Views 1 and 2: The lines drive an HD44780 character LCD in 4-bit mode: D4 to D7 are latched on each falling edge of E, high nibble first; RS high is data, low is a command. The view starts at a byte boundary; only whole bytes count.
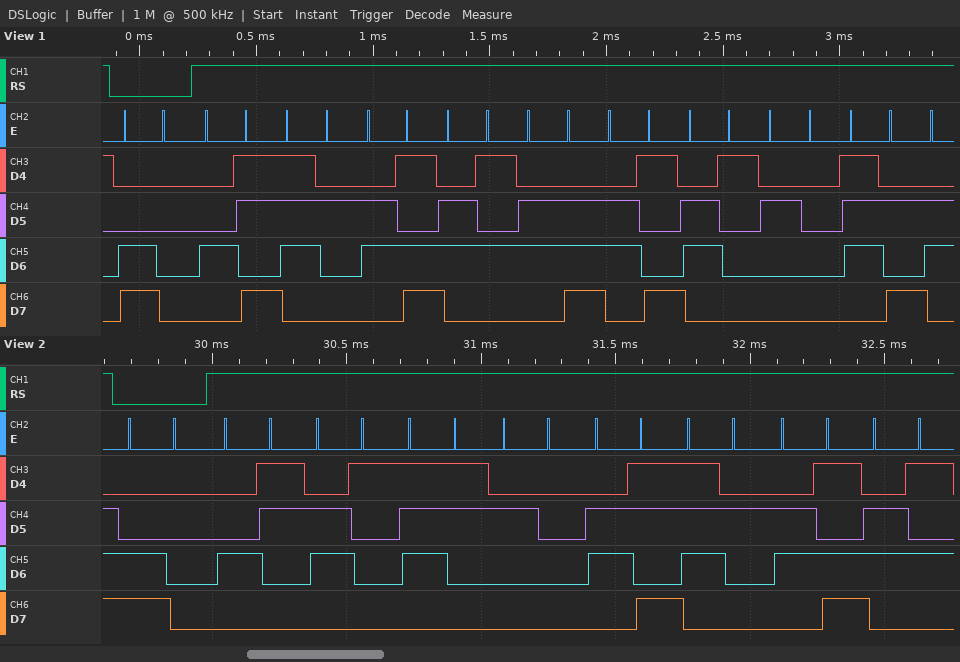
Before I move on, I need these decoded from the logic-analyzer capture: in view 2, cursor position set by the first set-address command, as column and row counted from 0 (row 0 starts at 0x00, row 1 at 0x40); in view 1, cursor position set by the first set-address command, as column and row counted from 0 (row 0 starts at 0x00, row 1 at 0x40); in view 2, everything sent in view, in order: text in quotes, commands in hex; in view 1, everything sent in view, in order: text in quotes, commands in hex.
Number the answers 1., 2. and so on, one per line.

1. column 0, row 1
2. column 0, row 1
3. 0xC0 "Cas krme"
4. 0xC0 "Krmenia z"
